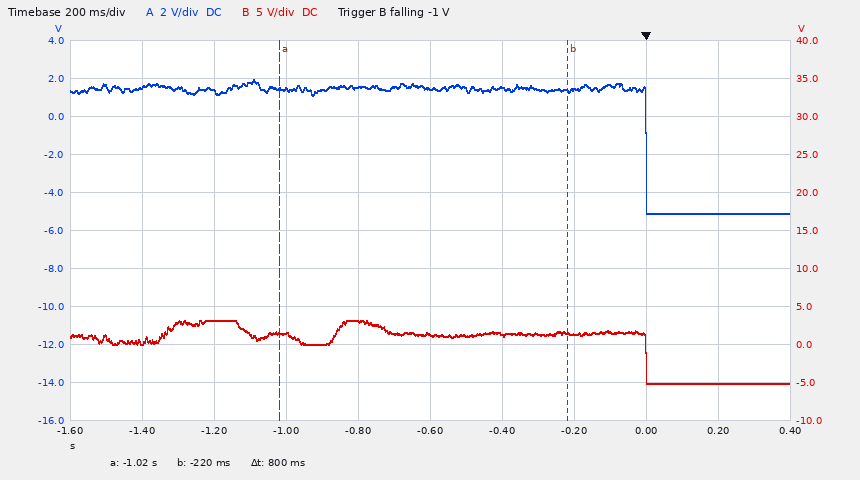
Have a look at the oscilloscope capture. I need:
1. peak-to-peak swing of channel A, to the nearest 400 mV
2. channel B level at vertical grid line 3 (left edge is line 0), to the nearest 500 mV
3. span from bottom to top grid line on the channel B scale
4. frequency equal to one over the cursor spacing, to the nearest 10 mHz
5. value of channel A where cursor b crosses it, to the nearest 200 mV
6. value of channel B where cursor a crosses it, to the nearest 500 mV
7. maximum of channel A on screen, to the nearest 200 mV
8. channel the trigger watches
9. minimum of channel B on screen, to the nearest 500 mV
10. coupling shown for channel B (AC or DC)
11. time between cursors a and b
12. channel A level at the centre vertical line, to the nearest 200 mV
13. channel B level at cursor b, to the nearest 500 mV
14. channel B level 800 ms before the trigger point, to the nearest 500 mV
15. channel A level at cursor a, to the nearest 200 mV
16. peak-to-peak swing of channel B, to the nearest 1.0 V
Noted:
7.2 V
1.5 V
50 V
1.25 Hz
1.4 V
1.5 V
2.0 V
channel B
-5.0 V
DC
800 ms
1.4 V
1.5 V
3.0 V
1.4 V
8.0 V
